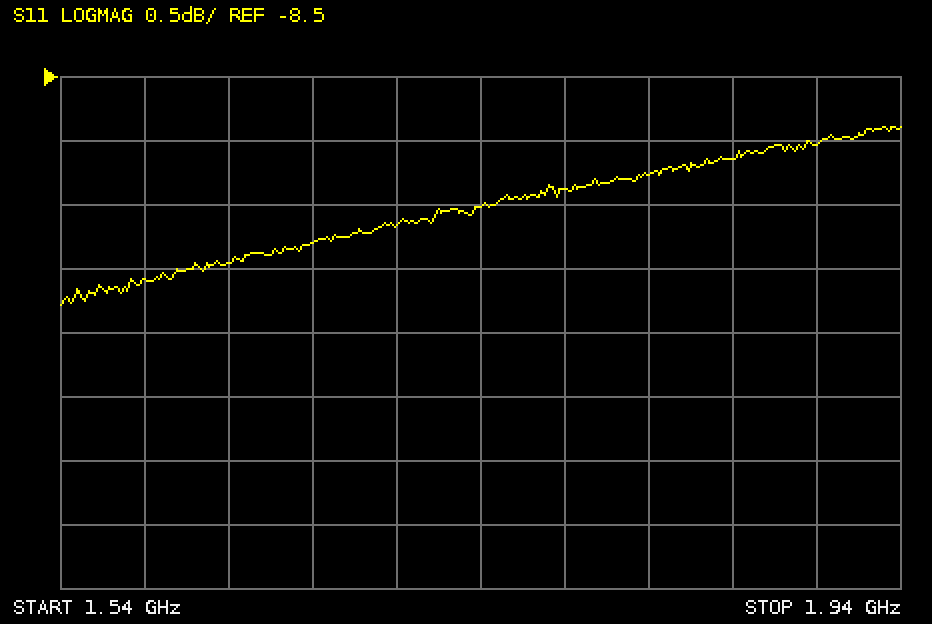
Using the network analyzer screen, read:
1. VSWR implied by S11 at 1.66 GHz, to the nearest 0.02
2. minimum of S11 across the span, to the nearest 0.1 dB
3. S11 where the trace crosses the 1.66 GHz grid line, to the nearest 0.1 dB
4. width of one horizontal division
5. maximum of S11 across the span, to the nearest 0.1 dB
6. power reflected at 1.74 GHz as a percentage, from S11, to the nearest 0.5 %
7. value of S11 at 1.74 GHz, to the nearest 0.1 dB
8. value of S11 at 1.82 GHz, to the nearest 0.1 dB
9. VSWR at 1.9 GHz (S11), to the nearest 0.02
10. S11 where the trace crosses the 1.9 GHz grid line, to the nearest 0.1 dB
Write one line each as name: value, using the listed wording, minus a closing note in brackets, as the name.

VSWR implied by S11 at 1.66 GHz, to the nearest 0.02: 1.96
minimum of S11 across the span, to the nearest 0.1 dB: -10.3 dB
S11 where the trace crosses the 1.66 GHz grid line, to the nearest 0.1 dB: -9.8 dB
width of one horizontal division: 40 MHz
maximum of S11 across the span, to the nearest 0.1 dB: -8.9 dB
power reflected at 1.74 GHz as a percentage, from S11, to the nearest 0.5 %: 11.0 %
value of S11 at 1.74 GHz, to the nearest 0.1 dB: -9.5 dB
value of S11 at 1.82 GHz, to the nearest 0.1 dB: -9.3 dB
VSWR at 1.9 GHz (S11), to the nearest 0.02: 2.10
S11 where the trace crosses the 1.9 GHz grid line, to the nearest 0.1 dB: -9.0 dB
